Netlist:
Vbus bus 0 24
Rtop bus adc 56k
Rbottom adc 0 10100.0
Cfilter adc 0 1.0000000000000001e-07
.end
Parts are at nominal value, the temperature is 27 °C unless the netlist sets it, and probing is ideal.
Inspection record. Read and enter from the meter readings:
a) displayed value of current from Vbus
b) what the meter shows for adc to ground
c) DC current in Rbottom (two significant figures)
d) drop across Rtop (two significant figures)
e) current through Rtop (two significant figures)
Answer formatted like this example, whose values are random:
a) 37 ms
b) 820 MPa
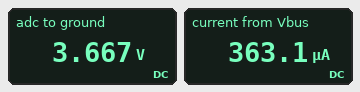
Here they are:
a) 363.1 µA
b) 3.667 V
c) 360 µA
d) 20 V
e) 360 µA
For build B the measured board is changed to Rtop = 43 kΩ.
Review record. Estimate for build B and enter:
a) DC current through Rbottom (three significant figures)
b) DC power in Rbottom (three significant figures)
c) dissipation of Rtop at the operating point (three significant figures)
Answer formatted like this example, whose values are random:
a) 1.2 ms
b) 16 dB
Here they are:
a) 452 µA
b) 2.06 mW
c) 8.78 mW
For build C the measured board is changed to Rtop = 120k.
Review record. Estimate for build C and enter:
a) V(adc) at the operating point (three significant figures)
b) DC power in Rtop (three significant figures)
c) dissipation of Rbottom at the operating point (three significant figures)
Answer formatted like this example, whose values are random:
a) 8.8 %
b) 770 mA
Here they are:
a) 1.86 V
b) 4.08 mW
c) 344 µW
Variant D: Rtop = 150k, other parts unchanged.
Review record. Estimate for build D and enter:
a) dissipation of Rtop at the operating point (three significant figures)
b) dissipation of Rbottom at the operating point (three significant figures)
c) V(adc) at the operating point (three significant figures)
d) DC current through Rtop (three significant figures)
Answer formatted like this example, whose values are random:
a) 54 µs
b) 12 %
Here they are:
a) 3.37 mW
b) 227 µW
c) 1.51 V
d) 150 µA
